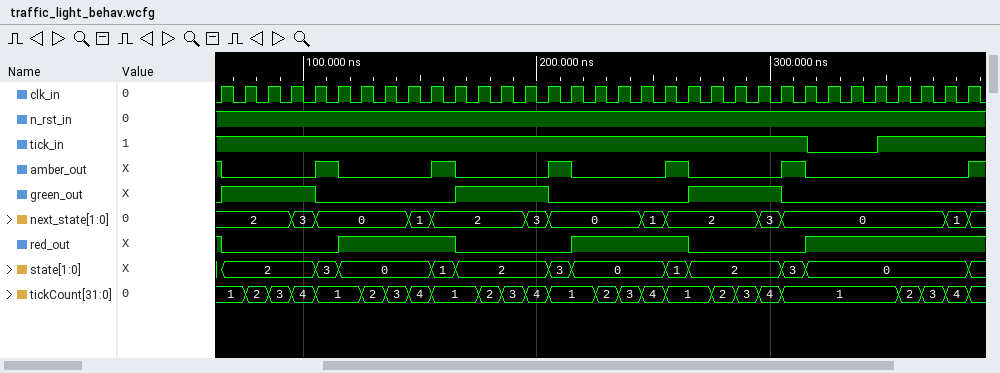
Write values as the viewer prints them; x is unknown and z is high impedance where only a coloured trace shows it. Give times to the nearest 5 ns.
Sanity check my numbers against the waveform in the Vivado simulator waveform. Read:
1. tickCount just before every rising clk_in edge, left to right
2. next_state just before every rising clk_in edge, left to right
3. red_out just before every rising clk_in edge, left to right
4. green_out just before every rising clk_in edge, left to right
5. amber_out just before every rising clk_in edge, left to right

1, 1, 2, 3, 4, 1, 1, 2, 3, 4, 1, 1, 2, 3, 4, 1, 1, 2, 3, 4, 1, 1, 2, 3, 4, 1, 1, 1, 1, 1, 2, 3, 4
2, 2, 2, 2, 3, 0, 0, 0, 0, 1, 2, 2, 2, 2, 3, 0, 0, 0, 0, 1, 2, 2, 2, 2, 3, 0, 0, 0, 0, 0, 0, 0, 1
1 0 0 0 0 0 1 1 1 1 1 0 0 0 0 0 1 1 1 1 1 0 0 0 0 0 1 1 1 1 1 1 1
0 1 1 1 1 0 0 0 0 0 0 1 1 1 1 0 0 0 0 0 0 1 1 1 1 0 0 0 0 0 0 0 0
1 0 0 0 0 1 0 0 0 0 1 0 0 0 0 1 0 0 0 0 1 0 0 0 0 1 0 0 0 0 0 0 0
